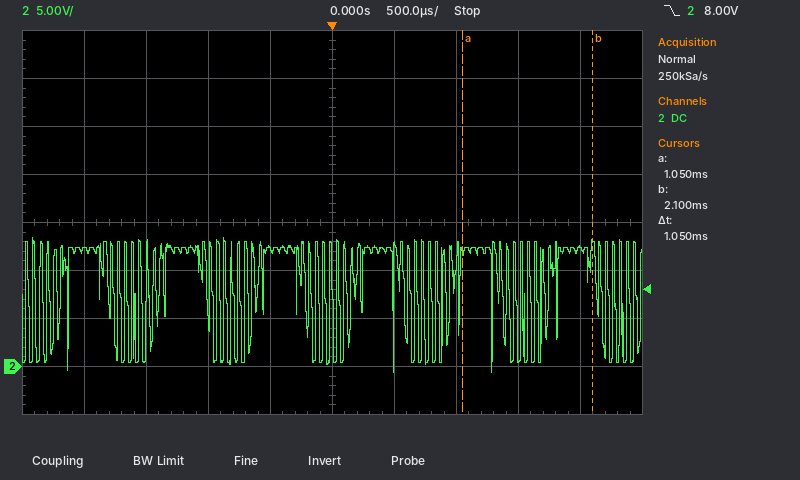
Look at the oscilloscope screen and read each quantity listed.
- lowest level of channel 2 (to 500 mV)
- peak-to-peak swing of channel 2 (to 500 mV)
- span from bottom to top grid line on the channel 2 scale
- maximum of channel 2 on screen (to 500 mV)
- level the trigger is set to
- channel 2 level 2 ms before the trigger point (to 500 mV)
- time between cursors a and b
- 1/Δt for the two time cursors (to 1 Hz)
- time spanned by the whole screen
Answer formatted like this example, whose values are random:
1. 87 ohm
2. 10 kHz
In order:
1. -500 mV
2. 14.0 V
3. 40 V
4. 13.5 V
5. 8.00 V
6. 12.0 V
7. 1.05 ms
8. 952 Hz
9. 5 ms
